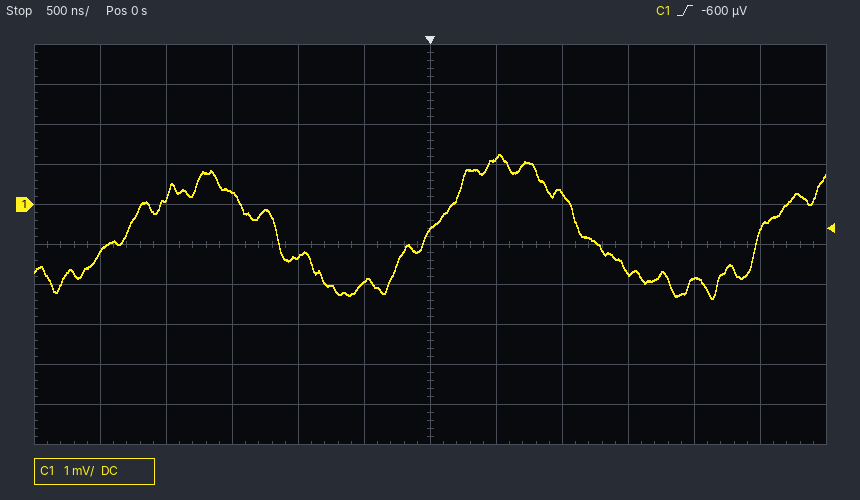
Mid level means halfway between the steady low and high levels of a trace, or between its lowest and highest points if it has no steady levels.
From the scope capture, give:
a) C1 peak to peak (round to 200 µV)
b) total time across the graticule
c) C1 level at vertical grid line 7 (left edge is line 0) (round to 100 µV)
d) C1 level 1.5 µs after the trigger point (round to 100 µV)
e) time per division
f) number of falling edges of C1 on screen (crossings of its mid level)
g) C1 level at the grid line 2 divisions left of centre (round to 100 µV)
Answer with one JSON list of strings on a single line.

["3.6 mV", "6 µs", "1.2 mV", "-1.7 mV", "500 ns", "2", "-1.3 mV"]
